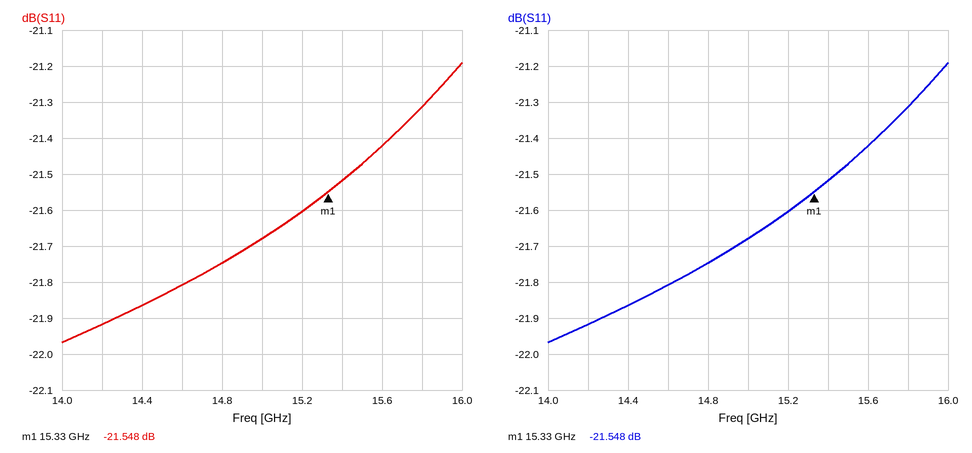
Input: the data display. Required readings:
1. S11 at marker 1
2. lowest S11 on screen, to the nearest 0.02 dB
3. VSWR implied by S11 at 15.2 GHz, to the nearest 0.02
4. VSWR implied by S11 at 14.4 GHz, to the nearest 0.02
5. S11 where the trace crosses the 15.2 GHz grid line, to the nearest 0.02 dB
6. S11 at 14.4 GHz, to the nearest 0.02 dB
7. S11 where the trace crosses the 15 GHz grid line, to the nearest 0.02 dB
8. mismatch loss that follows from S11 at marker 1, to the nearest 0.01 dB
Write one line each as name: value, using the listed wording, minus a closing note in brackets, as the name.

S11 at marker 1: -21.548 dB
lowest S11 on screen, to the nearest 0.02 dB: -21.96 dB
VSWR implied by S11 at 15.2 GHz, to the nearest 0.02: 1.18
VSWR implied by S11 at 14.4 GHz, to the nearest 0.02: 1.18
S11 where the trace crosses the 15.2 GHz grid line, to the nearest 0.02 dB: -21.60 dB
S11 at 14.4 GHz, to the nearest 0.02 dB: -21.86 dB
S11 where the trace crosses the 15 GHz grid line, to the nearest 0.02 dB: -21.68 dB
mismatch loss that follows from S11 at marker 1, to the nearest 0.01 dB: 0.03 dB
